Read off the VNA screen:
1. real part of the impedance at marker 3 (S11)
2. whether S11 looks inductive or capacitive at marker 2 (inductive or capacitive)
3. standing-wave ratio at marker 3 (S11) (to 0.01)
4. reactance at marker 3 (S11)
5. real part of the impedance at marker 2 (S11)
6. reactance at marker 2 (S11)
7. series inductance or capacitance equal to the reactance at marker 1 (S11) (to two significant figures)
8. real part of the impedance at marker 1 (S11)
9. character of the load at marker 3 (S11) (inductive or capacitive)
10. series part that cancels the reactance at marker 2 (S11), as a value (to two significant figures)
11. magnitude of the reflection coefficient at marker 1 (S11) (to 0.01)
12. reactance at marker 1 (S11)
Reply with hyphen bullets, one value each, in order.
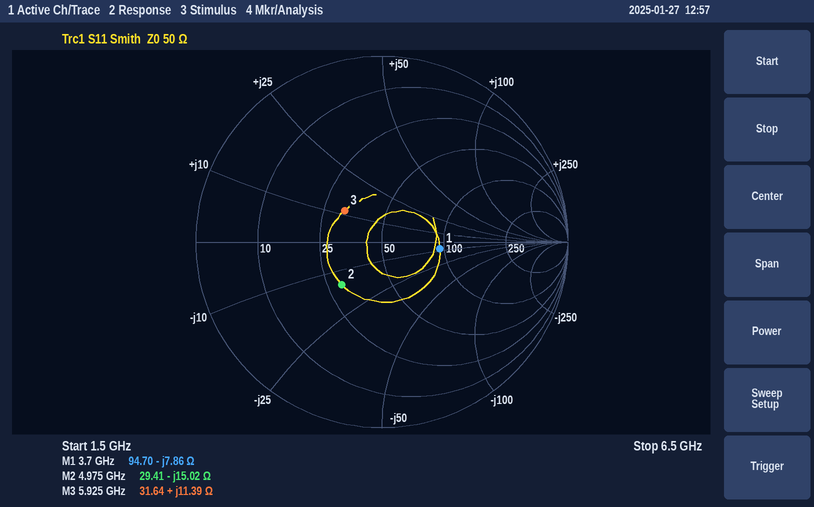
- 31.64 Ω
- capacitive
- 1.71
- +11.39 Ω
- 29.41 Ω
- -15.02 Ω
- 5.5 pF
- 94.70 Ω
- inductive
- 480 pH
- 0.31
- -7.86 Ω
